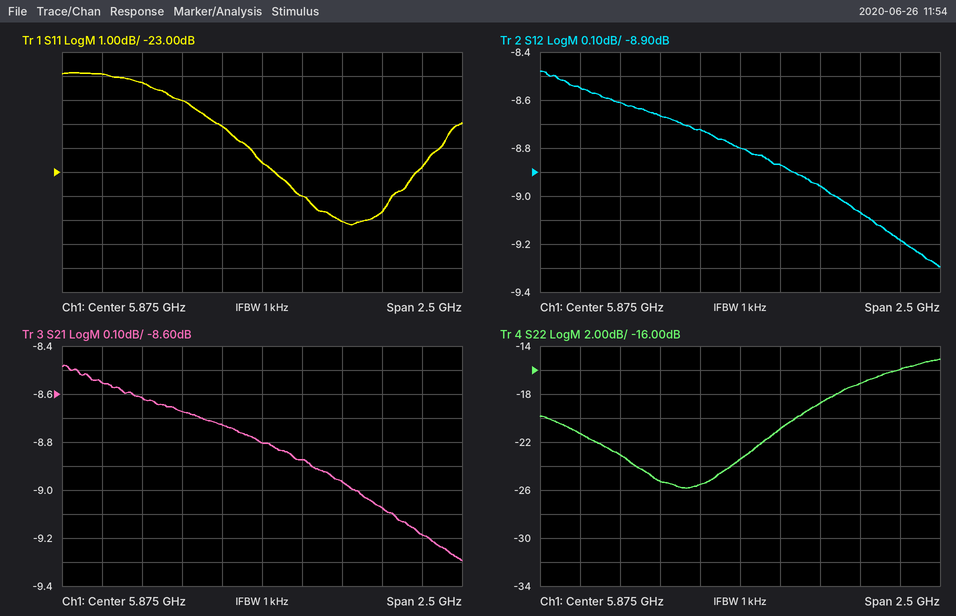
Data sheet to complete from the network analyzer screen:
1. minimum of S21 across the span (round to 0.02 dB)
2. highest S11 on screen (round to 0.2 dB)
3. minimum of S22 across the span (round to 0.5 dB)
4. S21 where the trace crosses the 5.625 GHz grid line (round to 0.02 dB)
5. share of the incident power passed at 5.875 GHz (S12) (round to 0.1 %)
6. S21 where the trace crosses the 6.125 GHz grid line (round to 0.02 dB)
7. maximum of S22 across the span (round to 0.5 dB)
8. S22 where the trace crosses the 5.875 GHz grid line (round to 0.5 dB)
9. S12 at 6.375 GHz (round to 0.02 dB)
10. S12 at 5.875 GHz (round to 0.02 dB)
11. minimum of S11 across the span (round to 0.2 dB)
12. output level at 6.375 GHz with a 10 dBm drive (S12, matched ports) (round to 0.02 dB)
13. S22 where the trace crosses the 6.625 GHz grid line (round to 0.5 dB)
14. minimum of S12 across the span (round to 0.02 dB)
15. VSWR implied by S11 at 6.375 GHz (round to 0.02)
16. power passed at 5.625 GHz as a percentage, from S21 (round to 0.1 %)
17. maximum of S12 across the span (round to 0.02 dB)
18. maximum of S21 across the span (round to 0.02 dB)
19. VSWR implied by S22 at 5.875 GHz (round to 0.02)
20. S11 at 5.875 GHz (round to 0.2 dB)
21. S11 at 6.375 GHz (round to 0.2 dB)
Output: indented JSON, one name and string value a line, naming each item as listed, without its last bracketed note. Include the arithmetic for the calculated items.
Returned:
{
  "minimum of S21 across the span": "-9.30 dB",
  "highest S11 on screen": "-18.8 dB",
  "minimum of S22 across the span": "-26.0 dB",
  "S21 where the trace crosses the 5.625 GHz grid line": "-8.72 dB",
  "share of the incident power passed at 5.875 GHz (S12)": "10^(-8.8/10) ≈ 13.2 %",
  "S21 where the trace crosses the 6.125 GHz grid line": "-8.88 dB",
  "maximum of S22 across the span": "-15.0 dB",
  "S22 where the trace crosses the 5.875 GHz grid line": "-23.5 dB",
  "S12 at 6.375 GHz": "-8.96 dB",
  "S12 at 5.875 GHz": "-8.80 dB",
  "minimum of S11 across the span": "-25.2 dB",
  "output level at 6.375 GHz with a 10 dBm drive (S12, matched ports)": "10 dBm + (-8.96 dB) = 1.04 dBm",
  "S22 where the trace crosses the 6.625 GHz grid line": "-17.0 dB",
  "minimum of S12 across the span": "-9.30 dB",
  "VSWR implied by S11 at 6.375 GHz": "|Γ| = 10^(-25/20) = 0.0562; VSWR = (1 + 0.0562)/(1 − 0.0562) ≈ 1.12",
  "power passed at 5.625 GHz as a percentage, from S21": "10^(-8.72/10) ≈ 13.4 %",
  "maximum of S12 across the span": "-8.48 dB",
  "maximum of S21 across the span": "-8.48 dB",
  "VSWR implied by S22 at 5.875 GHz": "|Γ| = 10^(-23.5/20) = 0.0668; VSWR = (1 + 0.0668)/(1 − 0.0668) ≈ 1.14",
  "S11 at 5.875 GHz": "-22.6 dB",
  "S11 at 6.375 GHz": "-25.0 dB"
}
